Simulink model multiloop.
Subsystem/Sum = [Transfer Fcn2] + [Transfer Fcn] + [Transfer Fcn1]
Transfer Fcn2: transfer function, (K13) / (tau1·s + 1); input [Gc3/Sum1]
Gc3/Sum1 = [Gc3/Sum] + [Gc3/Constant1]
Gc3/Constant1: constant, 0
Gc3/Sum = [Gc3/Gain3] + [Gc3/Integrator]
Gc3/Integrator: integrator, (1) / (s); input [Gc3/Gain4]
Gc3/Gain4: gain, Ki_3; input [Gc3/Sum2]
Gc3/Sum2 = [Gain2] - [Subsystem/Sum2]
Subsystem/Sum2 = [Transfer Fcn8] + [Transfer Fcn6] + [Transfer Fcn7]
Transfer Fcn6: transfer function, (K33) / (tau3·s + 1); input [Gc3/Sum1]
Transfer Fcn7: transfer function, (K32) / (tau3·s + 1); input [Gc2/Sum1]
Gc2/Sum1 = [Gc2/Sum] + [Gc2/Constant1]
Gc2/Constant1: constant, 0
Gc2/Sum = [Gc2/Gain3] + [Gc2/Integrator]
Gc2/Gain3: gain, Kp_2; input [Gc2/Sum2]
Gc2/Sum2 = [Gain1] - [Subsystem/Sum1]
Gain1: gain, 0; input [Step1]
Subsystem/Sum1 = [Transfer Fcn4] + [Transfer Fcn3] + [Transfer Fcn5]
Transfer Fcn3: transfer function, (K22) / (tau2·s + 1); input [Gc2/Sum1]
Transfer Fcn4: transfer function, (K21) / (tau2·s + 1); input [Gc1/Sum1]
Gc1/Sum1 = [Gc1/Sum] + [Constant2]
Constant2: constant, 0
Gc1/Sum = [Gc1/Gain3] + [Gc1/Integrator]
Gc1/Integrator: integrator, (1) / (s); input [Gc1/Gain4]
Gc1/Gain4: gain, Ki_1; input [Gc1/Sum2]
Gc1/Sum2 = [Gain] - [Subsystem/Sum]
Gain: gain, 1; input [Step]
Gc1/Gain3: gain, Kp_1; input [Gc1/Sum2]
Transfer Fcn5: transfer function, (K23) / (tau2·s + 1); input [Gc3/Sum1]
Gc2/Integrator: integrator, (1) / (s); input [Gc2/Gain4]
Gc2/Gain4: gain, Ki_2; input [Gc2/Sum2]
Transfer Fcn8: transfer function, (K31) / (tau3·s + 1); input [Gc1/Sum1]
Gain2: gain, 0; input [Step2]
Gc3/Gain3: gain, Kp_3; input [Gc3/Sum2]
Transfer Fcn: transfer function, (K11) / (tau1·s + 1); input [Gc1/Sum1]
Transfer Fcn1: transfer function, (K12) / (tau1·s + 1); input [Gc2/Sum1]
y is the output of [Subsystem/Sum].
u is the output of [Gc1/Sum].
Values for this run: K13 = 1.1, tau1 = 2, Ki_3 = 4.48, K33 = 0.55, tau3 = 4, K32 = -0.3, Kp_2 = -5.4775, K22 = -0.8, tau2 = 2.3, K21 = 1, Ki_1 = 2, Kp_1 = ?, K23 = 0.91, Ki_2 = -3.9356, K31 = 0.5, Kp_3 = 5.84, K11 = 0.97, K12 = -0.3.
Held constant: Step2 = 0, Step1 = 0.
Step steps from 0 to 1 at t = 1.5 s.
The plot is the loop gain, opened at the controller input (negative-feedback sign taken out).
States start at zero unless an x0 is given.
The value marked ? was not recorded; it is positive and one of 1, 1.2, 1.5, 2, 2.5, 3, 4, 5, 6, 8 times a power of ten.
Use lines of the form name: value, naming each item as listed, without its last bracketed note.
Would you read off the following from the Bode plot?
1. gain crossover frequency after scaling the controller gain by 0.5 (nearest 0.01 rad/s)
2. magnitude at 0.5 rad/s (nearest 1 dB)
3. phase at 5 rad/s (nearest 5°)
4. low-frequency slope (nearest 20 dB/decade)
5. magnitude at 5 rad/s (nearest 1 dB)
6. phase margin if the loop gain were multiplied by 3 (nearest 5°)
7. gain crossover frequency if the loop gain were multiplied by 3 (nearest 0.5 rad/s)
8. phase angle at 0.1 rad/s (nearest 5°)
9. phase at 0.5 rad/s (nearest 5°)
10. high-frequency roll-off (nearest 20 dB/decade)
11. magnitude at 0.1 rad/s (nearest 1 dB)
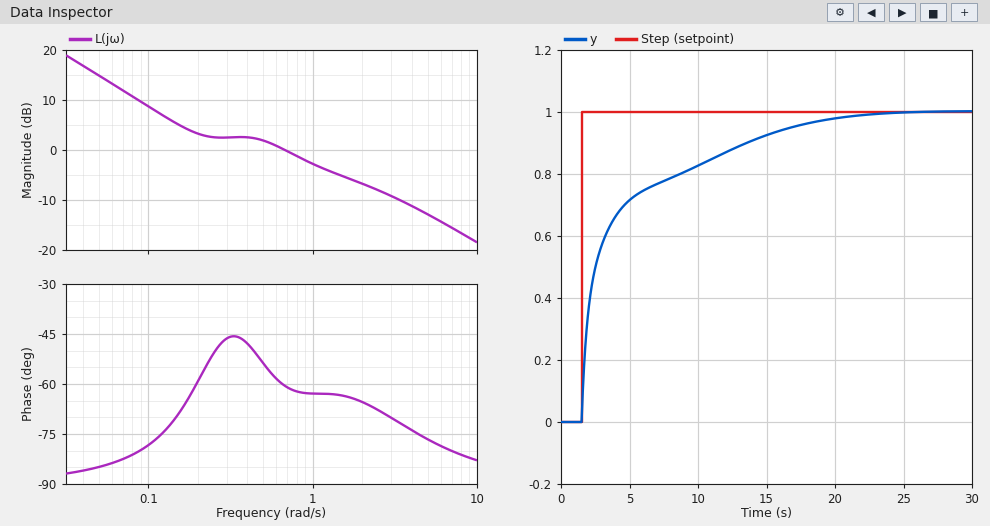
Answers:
gain crossover frequency after scaling the controller gain by 0.5: 0.14 rad/s
magnitude at 0.5 rad/s: 2 dB
phase at 5 rad/s: -75°
low-frequency slope: -20 dB/decade
magnitude at 5 rad/s: -13 dB
phase margin if the loop gain were multiplied by 3: 110°
gain crossover frequency if the loop gain were multiplied by 3: 3.0 rad/s
phase angle at 0.1 rad/s: -80°
phase at 0.5 rad/s: -55°
high-frequency roll-off: -20 dB/decade
magnitude at 0.1 rad/s: 9 dB
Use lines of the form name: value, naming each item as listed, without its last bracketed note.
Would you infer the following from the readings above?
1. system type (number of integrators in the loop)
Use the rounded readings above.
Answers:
system type: 1
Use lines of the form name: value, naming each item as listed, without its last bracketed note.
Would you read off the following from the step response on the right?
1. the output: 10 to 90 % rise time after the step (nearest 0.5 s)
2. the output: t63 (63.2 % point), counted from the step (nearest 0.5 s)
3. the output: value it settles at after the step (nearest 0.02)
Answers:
the output: 10 to 90 % rise time after the step: 12.0 s
the output: t63 (63.2 % point), counted from the step: 2.0 s
the output: value it settles at after the step: 1.00
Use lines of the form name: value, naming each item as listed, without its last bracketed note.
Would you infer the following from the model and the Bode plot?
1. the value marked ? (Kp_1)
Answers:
the value marked ?: 2.5
